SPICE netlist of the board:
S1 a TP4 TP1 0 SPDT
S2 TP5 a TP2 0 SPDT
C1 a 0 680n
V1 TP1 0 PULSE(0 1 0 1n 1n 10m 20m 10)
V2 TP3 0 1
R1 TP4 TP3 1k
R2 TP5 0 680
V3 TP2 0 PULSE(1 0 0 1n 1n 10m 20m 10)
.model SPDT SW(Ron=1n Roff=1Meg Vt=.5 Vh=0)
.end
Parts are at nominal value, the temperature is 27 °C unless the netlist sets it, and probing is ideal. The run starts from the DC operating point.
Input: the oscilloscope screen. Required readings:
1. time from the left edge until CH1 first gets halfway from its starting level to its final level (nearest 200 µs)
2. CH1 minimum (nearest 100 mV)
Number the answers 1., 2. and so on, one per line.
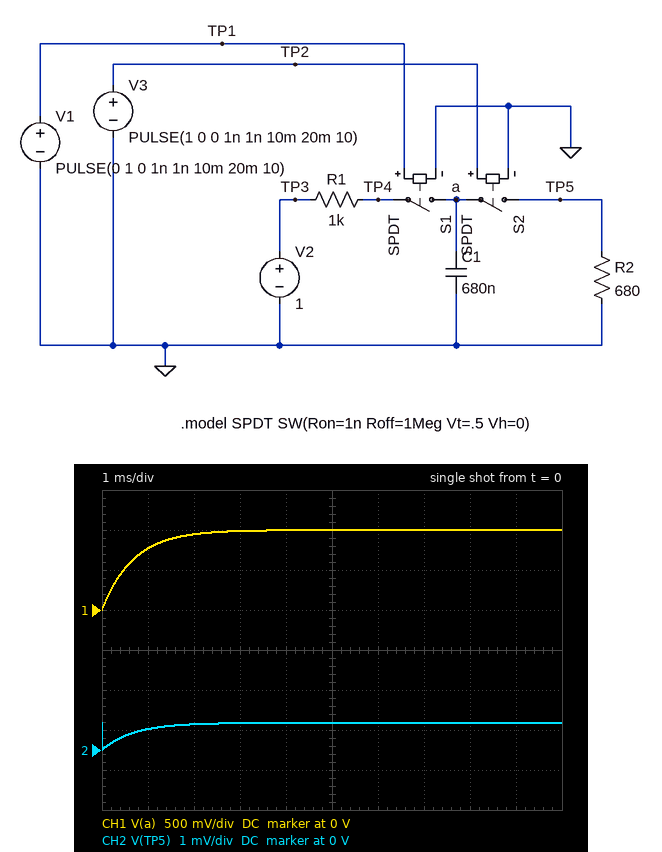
1. 400 µs
2. 0 V
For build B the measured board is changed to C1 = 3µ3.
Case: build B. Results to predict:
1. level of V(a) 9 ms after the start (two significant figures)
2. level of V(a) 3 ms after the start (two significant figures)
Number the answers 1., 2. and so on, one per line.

1. 930 mV
2. 600 mV
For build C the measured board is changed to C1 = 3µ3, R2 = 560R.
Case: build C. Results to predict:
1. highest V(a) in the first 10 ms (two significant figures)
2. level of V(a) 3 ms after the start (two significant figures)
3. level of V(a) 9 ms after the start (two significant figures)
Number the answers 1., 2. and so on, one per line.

1. 950 mV
2. 600 mV
3. 930 mV
